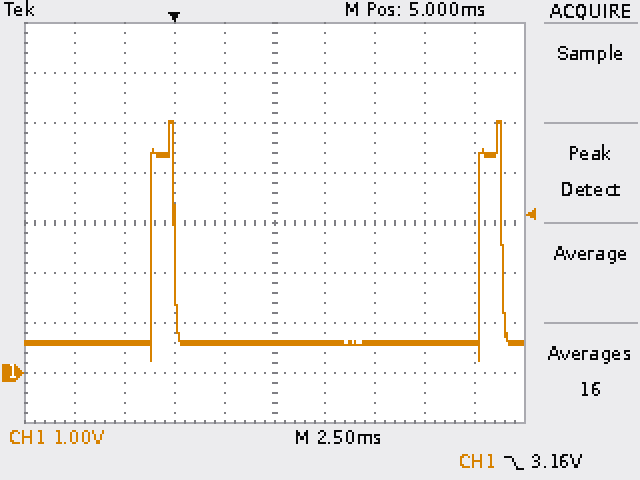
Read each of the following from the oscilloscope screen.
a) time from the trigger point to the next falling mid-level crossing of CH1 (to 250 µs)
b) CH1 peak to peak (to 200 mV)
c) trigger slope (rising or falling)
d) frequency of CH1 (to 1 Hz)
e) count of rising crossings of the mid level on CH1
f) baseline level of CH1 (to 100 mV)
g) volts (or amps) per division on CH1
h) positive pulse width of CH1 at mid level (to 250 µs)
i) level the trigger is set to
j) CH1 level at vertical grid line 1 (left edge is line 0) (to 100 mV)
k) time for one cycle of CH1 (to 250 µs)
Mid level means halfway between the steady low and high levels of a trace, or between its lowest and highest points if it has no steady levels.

16.50 ms
4.8 V
falling
61 Hz
2
600 mV
1 V
1.25 ms
3.16 V
600 mV
16.50 ms
